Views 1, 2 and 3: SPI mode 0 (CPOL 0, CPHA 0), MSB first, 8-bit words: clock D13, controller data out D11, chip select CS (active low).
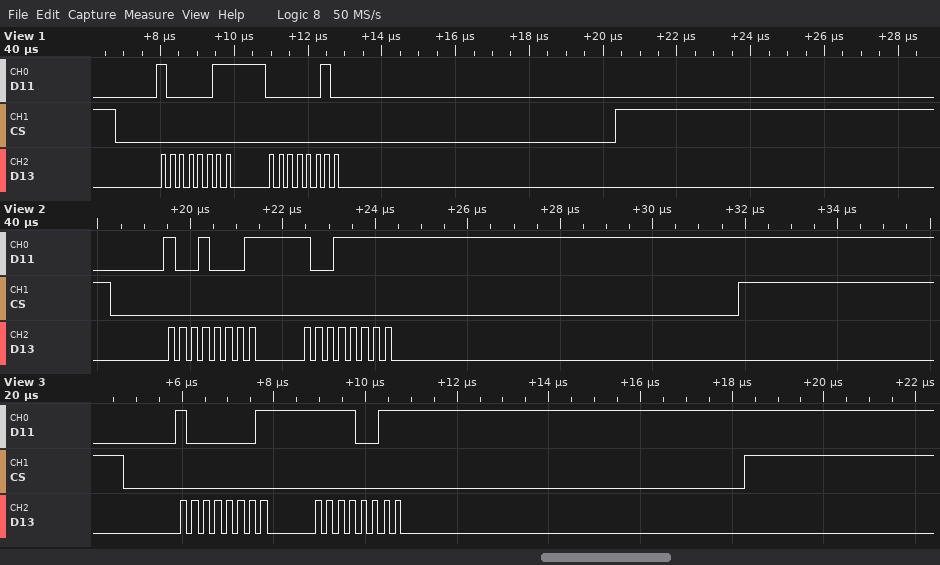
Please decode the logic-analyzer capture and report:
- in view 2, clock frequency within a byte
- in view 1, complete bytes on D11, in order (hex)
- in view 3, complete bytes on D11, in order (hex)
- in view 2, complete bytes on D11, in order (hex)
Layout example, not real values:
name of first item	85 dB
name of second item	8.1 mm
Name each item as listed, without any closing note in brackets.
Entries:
in view 2, clock frequency within a byte	4 MHz
in view 1, complete bytes on D11, in order	0x83 0x02
in view 3, complete bytes on D11, in order	81 F3
in view 2, complete bytes on D11, in order	91 9F
